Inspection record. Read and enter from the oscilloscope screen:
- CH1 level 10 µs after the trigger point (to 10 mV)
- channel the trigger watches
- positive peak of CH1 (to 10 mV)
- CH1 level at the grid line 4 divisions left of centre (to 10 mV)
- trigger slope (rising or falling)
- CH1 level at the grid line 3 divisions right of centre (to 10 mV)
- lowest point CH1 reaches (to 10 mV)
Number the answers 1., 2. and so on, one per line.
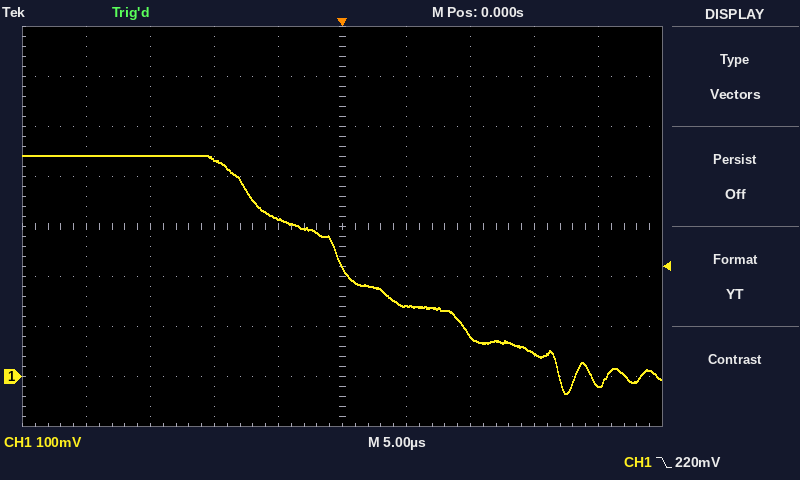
1. 80 mV
2. CH1
3. 440 mV
4. 440 mV
5. falling
6. 50 mV
7. -30 mV
